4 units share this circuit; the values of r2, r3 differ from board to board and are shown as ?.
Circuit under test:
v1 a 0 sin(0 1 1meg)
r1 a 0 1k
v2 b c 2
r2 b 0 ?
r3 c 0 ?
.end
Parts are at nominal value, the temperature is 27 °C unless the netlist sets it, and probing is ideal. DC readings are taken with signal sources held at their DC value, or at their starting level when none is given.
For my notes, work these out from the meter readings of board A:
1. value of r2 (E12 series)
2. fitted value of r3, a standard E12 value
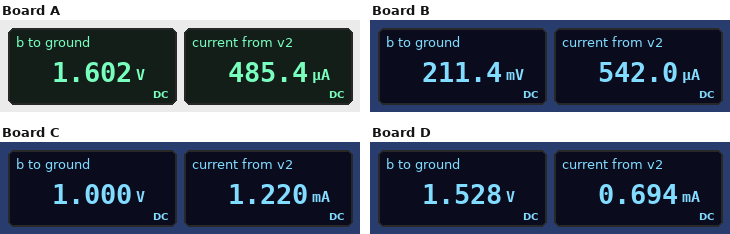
3.3 kΩ
820 Ω
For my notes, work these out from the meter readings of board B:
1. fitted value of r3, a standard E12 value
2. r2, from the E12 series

3.3 kΩ
390 Ω
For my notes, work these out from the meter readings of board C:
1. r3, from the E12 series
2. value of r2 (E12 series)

820 Ω
820 Ω
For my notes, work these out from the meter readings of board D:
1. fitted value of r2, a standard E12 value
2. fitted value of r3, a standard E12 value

2.2 kΩ
680 Ω
